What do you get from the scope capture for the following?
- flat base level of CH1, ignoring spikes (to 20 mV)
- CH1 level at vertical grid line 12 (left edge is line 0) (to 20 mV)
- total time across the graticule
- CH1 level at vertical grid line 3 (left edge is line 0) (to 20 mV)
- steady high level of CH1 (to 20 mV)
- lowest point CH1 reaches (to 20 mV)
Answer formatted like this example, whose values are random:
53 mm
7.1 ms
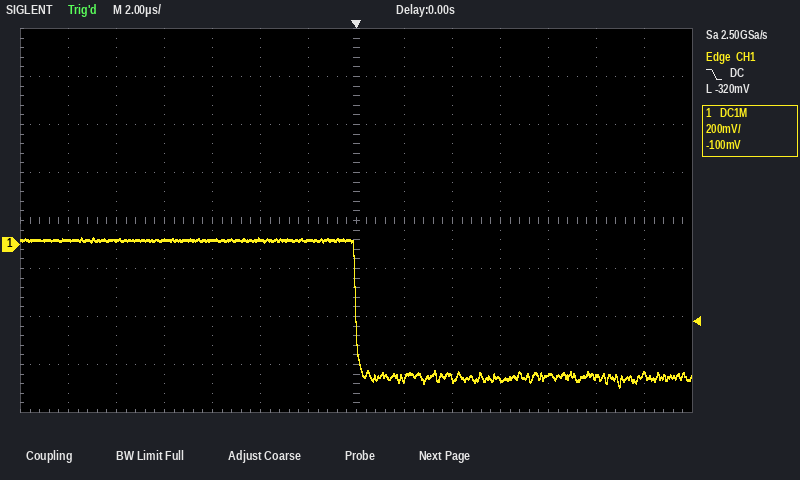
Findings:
-560 mV
-560 mV
28 µs
20 mV
20 mV
-600 mV
